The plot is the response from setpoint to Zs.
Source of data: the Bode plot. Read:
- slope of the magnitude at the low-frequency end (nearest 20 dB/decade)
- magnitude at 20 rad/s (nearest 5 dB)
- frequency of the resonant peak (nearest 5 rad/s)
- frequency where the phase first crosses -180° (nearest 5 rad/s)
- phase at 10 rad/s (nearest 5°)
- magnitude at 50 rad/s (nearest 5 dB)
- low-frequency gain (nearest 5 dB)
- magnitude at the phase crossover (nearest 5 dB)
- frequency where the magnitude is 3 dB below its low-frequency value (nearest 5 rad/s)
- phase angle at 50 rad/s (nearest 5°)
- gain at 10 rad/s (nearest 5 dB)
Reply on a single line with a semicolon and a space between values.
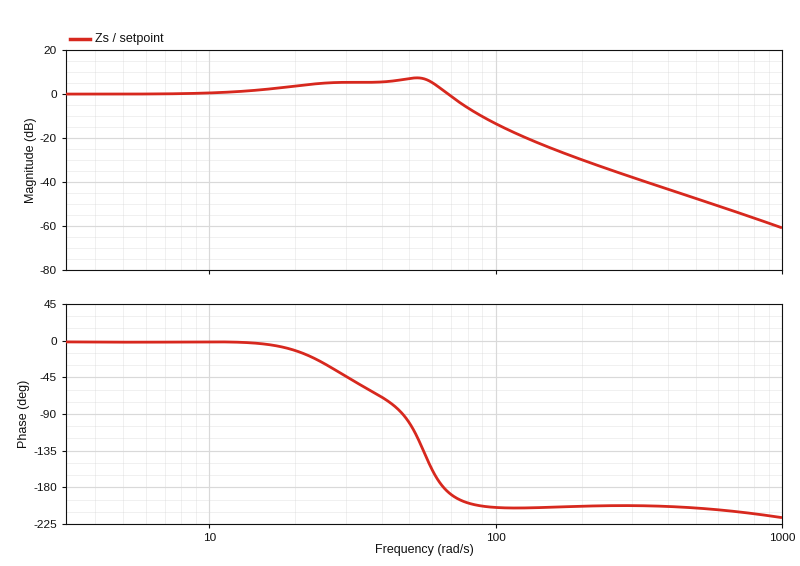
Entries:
0 dB/decade; 5 dB; 55 rad/s; 65 rad/s; 0°; 5 dB; 0 dB; 0 dB; 75 rad/s; -100°; 0 dB
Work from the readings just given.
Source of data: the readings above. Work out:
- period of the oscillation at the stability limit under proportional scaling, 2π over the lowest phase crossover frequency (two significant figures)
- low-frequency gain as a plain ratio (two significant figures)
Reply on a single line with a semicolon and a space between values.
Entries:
0.097 s; 1.0
